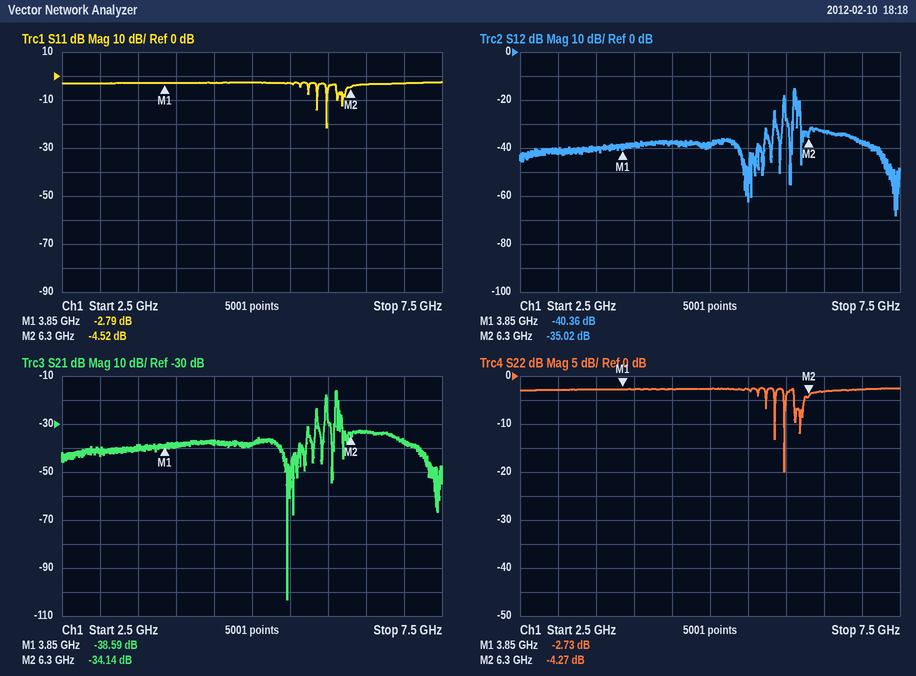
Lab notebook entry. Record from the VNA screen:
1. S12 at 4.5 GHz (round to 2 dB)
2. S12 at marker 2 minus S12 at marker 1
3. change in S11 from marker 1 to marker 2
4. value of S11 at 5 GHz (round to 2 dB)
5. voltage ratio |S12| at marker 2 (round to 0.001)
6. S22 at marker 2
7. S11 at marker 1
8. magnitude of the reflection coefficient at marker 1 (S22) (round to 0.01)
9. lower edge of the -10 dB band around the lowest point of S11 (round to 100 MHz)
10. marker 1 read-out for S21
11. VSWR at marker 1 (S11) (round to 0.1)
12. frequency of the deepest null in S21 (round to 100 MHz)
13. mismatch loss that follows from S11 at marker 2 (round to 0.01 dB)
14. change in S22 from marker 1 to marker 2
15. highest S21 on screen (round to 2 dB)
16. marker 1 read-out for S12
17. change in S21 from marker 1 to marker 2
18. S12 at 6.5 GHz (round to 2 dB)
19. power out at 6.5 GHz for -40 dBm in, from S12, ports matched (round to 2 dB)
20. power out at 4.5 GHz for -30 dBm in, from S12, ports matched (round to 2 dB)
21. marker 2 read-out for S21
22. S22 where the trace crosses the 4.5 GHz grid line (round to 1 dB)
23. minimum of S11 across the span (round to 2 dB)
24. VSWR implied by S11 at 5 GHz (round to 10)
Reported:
-38 dB
5.34 dB
-1.73 dB
-2 dB
0.018
-4.27 dB
-2.79 dB
0.73
6.0 GHz
-38.59 dB
6.3
5.5 GHz
1.89 dB
-1.54 dB
-16 dB
-40.36 dB
4.45 dB
-34 dB
-74 dBm
-68 dBm
-34.14 dB
-3 dB
-22 dB
10
